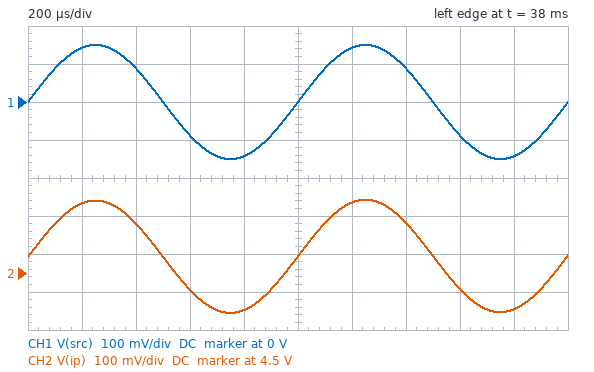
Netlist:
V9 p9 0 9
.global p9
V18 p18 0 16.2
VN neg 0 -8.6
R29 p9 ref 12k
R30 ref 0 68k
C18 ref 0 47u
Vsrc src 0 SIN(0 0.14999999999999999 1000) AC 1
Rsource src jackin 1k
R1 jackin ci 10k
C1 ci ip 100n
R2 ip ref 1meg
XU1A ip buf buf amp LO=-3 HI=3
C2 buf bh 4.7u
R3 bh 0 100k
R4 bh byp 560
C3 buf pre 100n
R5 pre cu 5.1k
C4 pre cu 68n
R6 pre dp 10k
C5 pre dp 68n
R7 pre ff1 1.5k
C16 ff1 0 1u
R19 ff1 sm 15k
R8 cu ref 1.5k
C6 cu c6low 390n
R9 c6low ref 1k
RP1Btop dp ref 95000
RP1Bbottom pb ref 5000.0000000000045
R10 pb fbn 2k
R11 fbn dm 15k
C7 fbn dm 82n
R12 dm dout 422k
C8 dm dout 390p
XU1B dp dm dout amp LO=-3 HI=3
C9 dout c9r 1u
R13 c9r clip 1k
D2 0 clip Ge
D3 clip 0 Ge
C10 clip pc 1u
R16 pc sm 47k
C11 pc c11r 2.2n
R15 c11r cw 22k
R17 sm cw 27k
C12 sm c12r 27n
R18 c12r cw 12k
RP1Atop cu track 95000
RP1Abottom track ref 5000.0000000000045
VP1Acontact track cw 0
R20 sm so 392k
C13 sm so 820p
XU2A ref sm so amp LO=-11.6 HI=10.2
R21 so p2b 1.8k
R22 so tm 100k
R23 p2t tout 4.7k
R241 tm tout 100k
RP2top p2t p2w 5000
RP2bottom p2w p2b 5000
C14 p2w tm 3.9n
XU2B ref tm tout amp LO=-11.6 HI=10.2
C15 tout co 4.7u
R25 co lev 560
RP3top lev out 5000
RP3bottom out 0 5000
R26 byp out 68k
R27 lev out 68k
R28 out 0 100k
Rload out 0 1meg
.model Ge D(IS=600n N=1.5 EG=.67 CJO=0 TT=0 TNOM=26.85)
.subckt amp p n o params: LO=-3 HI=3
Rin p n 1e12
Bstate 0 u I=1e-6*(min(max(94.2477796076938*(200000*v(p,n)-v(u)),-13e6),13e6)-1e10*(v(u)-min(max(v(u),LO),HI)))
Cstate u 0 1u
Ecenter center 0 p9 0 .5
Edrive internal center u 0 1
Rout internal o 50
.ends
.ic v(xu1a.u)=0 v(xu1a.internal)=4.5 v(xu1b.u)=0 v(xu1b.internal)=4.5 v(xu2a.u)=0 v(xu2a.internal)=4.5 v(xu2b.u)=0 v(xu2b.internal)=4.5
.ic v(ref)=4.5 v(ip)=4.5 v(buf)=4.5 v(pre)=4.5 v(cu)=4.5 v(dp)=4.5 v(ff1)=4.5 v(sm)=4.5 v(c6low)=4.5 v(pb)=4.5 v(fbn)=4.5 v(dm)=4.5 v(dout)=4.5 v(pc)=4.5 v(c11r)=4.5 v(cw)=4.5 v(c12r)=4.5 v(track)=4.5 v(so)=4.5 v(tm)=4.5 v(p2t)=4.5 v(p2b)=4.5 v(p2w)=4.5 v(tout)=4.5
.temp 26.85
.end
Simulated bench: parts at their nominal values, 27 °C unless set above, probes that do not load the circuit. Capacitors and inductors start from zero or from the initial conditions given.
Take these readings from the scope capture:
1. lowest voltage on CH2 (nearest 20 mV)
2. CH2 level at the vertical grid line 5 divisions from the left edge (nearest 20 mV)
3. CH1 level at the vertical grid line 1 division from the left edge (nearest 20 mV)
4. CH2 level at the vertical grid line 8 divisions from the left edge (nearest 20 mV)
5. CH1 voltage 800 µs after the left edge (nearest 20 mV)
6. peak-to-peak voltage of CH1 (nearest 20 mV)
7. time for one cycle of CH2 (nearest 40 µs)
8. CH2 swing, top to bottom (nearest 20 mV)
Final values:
4.40 V
4.54 V
140 mV
4.46 V
-140 mV
300 mV
1.00 ms
300 mV
